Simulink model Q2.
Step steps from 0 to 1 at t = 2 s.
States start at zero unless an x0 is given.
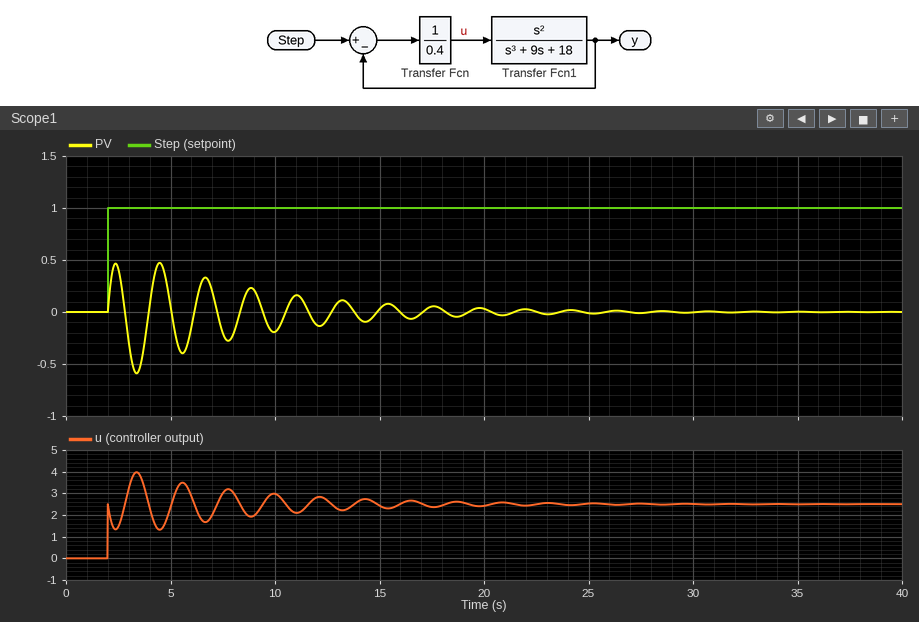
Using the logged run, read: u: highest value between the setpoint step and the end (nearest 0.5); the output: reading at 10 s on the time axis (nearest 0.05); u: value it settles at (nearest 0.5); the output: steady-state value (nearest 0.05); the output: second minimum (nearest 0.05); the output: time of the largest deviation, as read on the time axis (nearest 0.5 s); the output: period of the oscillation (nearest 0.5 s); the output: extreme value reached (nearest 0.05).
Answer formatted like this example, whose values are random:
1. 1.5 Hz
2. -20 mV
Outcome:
1. 4.0
2. -0.20
3. 2.5
4. 0.00
5. -0.40
6. 3.5 s
7. 2.0 s
8. -0.60
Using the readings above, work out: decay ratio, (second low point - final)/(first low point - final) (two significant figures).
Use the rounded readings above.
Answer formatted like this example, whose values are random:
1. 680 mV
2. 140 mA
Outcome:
1. 0.67
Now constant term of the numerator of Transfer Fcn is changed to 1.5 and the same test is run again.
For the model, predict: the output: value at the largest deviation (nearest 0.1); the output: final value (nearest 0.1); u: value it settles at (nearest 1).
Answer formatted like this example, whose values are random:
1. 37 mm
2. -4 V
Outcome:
1. 0.6
2. 0.0
3. 4
